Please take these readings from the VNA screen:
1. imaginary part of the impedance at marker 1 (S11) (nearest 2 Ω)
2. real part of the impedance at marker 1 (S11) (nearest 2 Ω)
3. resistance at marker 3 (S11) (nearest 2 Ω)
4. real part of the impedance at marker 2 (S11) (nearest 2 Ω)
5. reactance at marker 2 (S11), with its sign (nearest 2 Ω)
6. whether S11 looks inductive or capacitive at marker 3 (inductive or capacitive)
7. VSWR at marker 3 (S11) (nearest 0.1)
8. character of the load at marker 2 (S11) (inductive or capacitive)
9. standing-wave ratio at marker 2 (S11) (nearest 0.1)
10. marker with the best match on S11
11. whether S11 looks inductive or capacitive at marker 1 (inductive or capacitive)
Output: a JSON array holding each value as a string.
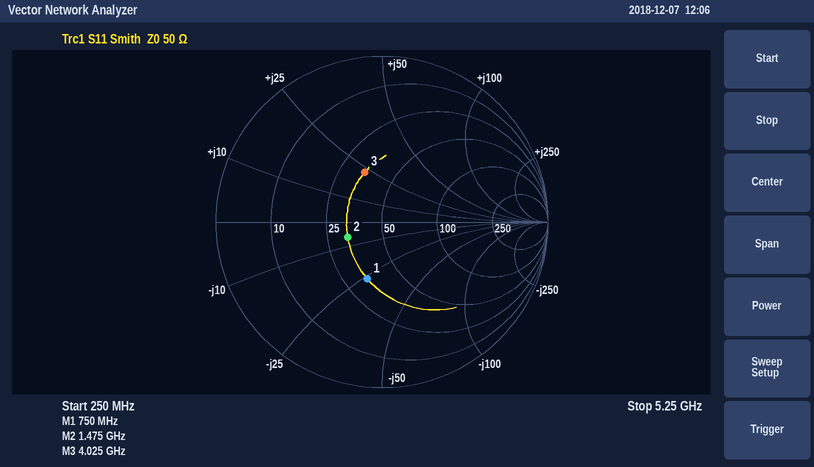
["-26 Ω", "34 Ω", "34 Ω", "32 Ω", "-6 Ω", "inductive", "1.9", "capacitive", "1.6", "marker 2", "capacitive"]
